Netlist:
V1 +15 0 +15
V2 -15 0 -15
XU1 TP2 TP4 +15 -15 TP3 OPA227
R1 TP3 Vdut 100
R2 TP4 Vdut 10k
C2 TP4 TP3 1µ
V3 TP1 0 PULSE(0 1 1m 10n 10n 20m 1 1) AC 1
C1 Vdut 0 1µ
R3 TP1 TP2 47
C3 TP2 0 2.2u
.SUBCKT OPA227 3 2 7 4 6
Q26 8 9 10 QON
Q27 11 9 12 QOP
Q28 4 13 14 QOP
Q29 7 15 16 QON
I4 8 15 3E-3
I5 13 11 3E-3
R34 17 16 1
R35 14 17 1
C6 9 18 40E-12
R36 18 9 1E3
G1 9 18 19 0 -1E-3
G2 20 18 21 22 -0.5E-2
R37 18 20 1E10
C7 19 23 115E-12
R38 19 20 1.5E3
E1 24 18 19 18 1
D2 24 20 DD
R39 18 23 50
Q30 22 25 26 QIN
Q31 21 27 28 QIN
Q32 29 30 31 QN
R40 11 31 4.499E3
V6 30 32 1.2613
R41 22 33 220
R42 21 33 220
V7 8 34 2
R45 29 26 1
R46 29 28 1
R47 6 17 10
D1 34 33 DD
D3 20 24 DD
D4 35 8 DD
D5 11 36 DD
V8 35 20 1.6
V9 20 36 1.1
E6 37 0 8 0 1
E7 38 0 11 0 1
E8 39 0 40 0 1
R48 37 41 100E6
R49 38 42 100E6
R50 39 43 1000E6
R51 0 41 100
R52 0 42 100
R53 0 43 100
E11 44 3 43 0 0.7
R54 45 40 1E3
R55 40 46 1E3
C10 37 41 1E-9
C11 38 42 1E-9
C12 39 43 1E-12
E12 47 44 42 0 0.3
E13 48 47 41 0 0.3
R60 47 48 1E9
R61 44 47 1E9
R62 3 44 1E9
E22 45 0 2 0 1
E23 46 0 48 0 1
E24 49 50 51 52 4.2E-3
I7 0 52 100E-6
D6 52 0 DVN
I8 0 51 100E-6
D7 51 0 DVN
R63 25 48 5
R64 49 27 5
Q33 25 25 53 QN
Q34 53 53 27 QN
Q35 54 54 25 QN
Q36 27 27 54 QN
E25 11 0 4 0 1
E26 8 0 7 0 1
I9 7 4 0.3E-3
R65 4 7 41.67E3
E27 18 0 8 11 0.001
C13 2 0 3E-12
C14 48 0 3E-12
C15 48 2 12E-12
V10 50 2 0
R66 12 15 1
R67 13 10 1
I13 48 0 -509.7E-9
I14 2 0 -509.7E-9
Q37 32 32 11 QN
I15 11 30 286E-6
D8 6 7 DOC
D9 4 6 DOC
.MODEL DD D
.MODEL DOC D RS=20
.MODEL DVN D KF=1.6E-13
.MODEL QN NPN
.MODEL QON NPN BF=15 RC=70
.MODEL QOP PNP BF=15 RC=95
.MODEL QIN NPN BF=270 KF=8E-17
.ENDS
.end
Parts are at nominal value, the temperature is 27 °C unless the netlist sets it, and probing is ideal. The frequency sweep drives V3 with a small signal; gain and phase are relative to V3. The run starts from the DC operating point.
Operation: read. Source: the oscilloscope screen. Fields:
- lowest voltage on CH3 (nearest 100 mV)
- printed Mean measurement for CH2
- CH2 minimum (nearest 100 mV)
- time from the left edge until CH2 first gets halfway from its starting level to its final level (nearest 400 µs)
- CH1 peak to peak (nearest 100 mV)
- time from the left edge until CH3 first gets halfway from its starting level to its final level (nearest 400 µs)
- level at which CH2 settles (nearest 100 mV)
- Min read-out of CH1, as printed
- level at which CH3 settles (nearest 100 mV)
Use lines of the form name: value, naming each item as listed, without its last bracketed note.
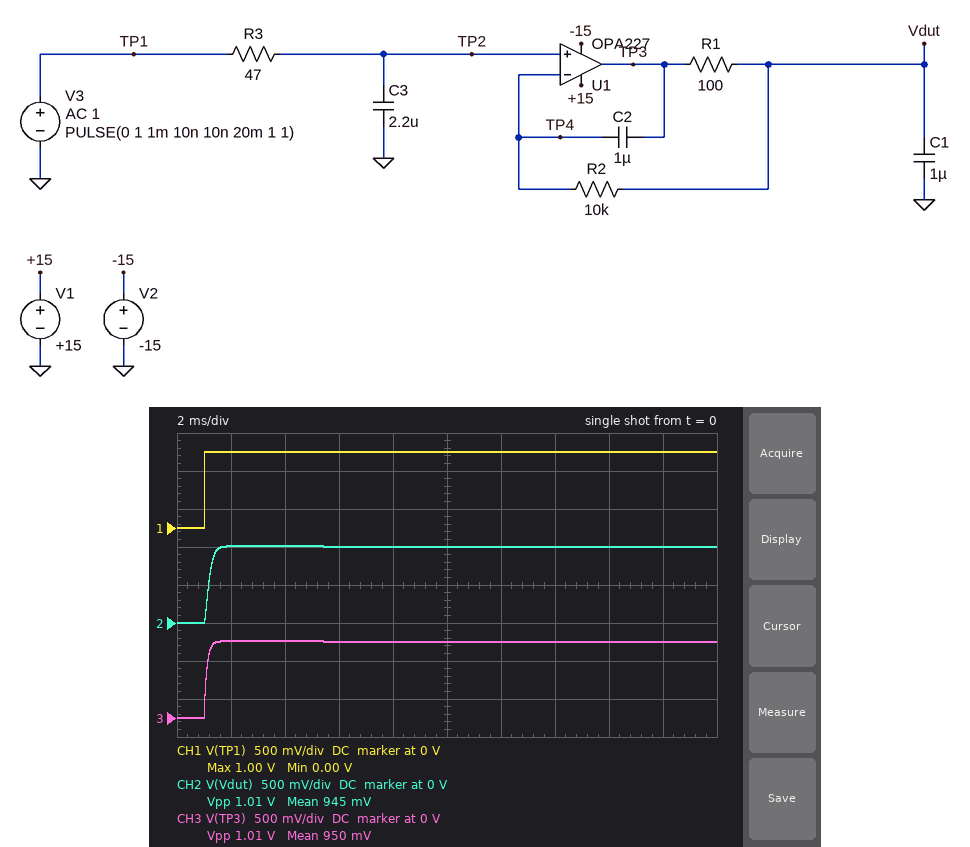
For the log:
lowest voltage on CH3: 0 V
printed Mean measurement for CH2: 945 mV
CH2 minimum: 0 V
time from the left edge until CH2 first gets halfway from its starting level to its final level: 1.2 ms
CH1 peak to peak: 1.0 V
time from the left edge until CH3 first gets halfway from its starting level to its final level: 1.2 ms
level at which CH2 settles: 1.0 V
Min read-out of CH1, as printed: 0.00 V
level at which CH3 settles: 1.0 V
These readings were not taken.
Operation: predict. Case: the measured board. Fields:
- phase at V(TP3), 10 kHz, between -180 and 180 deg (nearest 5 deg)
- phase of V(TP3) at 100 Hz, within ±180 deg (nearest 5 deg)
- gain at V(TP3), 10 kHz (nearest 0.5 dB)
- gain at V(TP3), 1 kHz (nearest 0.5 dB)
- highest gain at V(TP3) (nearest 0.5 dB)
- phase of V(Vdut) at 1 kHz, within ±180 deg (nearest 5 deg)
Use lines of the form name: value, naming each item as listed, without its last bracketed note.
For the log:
phase at V(TP3), 10 kHz, between -180 and 180 deg: -80 deg
phase of V(TP3) at 100 Hz, within ±180 deg: -5 deg
gain at V(TP3), 10 kHz: -16.5 dB
gain at V(TP3), 1 kHz: -1.5 dB
highest gain at V(TP3): 0 dB
phase of V(Vdut) at 1 kHz, within ±180 deg: -65 deg
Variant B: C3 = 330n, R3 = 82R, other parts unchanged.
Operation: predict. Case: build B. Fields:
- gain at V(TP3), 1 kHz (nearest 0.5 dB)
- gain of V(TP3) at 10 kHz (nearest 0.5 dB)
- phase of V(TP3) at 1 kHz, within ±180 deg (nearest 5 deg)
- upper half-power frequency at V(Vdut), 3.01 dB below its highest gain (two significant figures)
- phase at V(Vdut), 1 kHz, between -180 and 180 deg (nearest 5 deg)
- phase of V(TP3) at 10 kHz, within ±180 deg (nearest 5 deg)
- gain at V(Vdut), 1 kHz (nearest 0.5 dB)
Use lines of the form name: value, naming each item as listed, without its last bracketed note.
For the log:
gain at V(TP3), 1 kHz: 0 dB
gain of V(TP3) at 10 kHz: -6.0 dB
phase of V(TP3) at 1 kHz, within ±180 deg: -10 deg
upper half-power frequency at V(Vdut), 3.01 dB below its highest gain: 1.5 kHz
phase at V(Vdut), 1 kHz, between -180 and 180 deg: -40 deg
phase of V(TP3) at 10 kHz, within ±180 deg: -60 deg
gain at V(Vdut), 1 kHz: -1.5 dB
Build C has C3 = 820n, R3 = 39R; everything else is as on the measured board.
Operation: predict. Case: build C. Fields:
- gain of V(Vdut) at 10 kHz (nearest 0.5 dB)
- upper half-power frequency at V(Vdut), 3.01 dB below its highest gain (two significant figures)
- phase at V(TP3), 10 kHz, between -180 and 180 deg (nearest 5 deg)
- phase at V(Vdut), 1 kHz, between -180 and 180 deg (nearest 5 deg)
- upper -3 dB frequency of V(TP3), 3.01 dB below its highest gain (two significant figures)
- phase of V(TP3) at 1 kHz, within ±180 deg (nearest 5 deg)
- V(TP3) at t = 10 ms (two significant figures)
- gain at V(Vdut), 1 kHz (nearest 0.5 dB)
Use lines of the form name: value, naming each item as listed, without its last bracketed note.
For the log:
gain of V(Vdut) at 10 kHz: -23.0 dB
upper half-power frequency at V(Vdut), 3.01 dB below its highest gain: 1.5 kHz
phase at V(TP3), 10 kHz, between -180 and 180 deg: -65 deg
phase at V(Vdut), 1 kHz, between -180 and 180 deg: -45 deg
upper -3 dB frequency of V(TP3), 3.01 dB below its highest gain: 4.9 kHz
phase of V(TP3) at 1 kHz, within ±180 deg: -10 deg
V(TP3) at t = 10 ms: 1.0 V
gain at V(Vdut), 1 kHz: -1.5 dB
